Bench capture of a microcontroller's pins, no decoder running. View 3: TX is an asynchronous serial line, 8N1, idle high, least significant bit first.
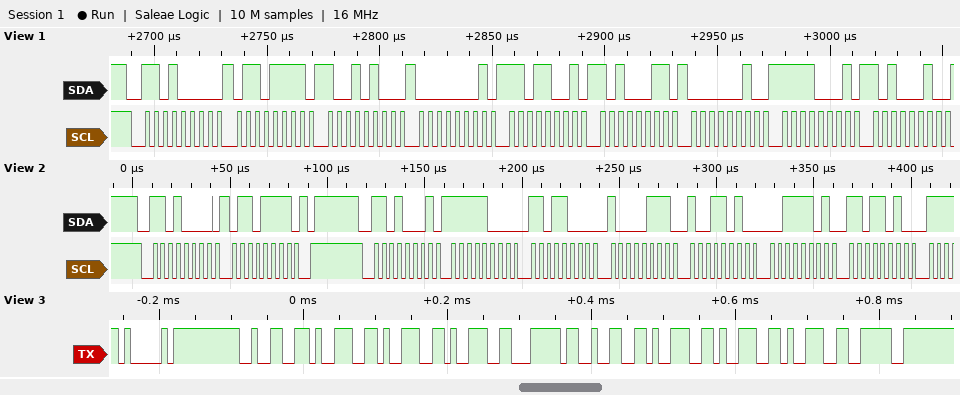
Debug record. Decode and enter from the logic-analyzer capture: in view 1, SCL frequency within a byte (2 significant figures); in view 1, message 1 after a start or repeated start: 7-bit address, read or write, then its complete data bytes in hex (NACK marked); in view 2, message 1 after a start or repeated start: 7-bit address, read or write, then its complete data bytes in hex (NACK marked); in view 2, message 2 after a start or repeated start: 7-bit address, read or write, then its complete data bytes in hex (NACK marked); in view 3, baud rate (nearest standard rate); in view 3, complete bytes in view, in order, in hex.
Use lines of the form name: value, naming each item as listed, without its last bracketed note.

in view 1, SCL frequency within a byte: 250 kHz
in view 1, message 1 after a start or repeated start: 7-bit address, read or write, then its complete data bytes in hex: 0x68 write: 6F 94 01 D9 A3 02 F1 A2
in view 2, message 1 after a start or repeated start: 7-bit address, read or write, then its complete data bytes in hex: 0x68 write: 6F
in view 2, message 2 after a start or repeated start: 7-bit address, read or write, then its complete data bytes in hex: 0x68 read: F8 D8 87 9A 3D DA
in view 3, baud rate: 115200 baud
in view 3, complete bytes in view, in order, in hex: 41 32 39 39 39 7C 32 39 39 39 3E
